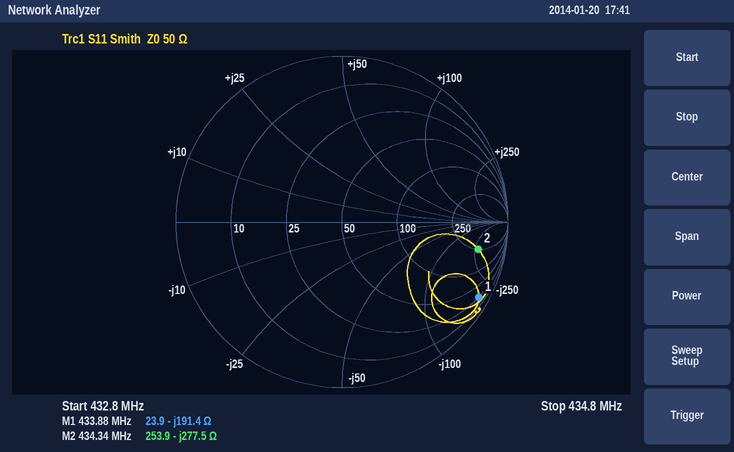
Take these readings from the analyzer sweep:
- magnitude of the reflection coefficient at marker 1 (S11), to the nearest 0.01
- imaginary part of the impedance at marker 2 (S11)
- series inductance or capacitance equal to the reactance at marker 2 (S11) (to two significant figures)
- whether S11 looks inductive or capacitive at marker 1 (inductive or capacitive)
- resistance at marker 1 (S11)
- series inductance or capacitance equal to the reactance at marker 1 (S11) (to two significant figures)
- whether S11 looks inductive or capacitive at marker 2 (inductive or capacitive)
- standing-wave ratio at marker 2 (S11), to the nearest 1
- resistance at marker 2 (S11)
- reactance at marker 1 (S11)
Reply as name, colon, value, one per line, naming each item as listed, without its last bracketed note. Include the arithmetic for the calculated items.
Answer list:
magnitude of the reflection coefficient at marker 1 (S11), to the nearest 0.01: 0.94
imaginary part of the impedance at marker 2: -277.5 Ω
series inductance or capacitance equal to the reactance at marker 2 (S11): C = 1/(2π × 434.34 MHz × 277.5 Ω) ≈ 1.3 pF
whether S11 looks inductive or capacitive at marker 1: capacitive
resistance at marker 1: 23.9 Ω
series inductance or capacitance equal to the reactance at marker 1 (S11): C = 1/(2π × 433.88 MHz × 191.4 Ω) ≈ 1.9 pF
whether S11 looks inductive or capacitive at marker 2: capacitive
standing-wave ratio at marker 2 (S11), to the nearest 1: 11
resistance at marker 2: 253.9 Ω
reactance at marker 1: -191.4 Ω
